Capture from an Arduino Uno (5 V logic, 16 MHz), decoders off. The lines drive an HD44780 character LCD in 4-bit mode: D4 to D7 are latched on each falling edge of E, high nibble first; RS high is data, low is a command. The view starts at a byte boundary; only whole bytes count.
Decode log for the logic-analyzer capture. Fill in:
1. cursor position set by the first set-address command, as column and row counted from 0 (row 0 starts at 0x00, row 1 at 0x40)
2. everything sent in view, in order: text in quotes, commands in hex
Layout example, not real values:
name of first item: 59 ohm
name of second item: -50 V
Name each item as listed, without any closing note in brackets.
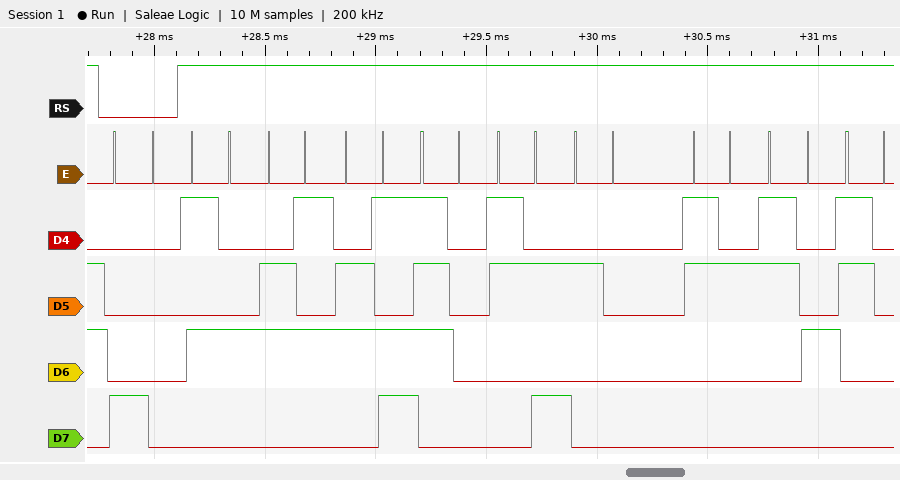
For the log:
cursor position set by the first set-address command, as column and row counted from 0: column 0, row 0
everything sent in view, in order: text in quotes, commands in hex: 0x80 "Temp: 240"
